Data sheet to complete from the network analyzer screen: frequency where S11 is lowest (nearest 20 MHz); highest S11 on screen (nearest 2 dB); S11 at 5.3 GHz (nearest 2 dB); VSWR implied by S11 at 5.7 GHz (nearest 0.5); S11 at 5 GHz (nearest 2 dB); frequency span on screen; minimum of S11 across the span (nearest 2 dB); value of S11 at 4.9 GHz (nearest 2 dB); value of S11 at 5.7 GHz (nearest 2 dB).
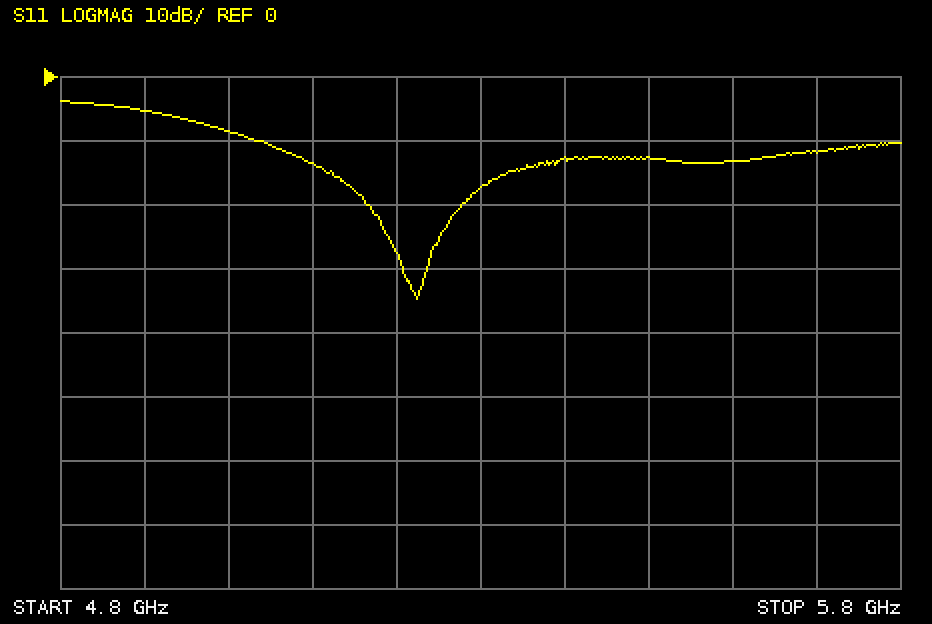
5.22 GHz
-4 dB
-18 dB
1.5
-8 dB
1 GHz
-34 dB
-6 dB
-12 dB
